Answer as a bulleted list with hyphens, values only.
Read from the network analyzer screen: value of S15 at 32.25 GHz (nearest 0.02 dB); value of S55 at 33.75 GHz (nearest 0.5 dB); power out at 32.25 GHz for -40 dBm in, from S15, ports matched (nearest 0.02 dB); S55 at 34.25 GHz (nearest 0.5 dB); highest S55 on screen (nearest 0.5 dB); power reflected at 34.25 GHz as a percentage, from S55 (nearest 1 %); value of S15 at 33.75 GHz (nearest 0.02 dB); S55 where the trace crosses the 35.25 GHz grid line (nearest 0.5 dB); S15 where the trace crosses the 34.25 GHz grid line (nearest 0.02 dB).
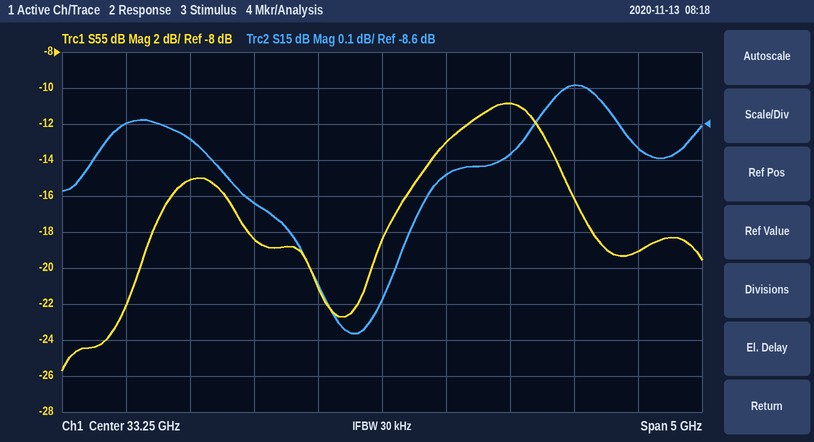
- -8.82 dB
- -13.0 dB
- -48.82 dBm
- -11.0 dB
- -11.0 dB
- 8 %
- -8.74 dB
- -19.0 dB
- -8.68 dB
